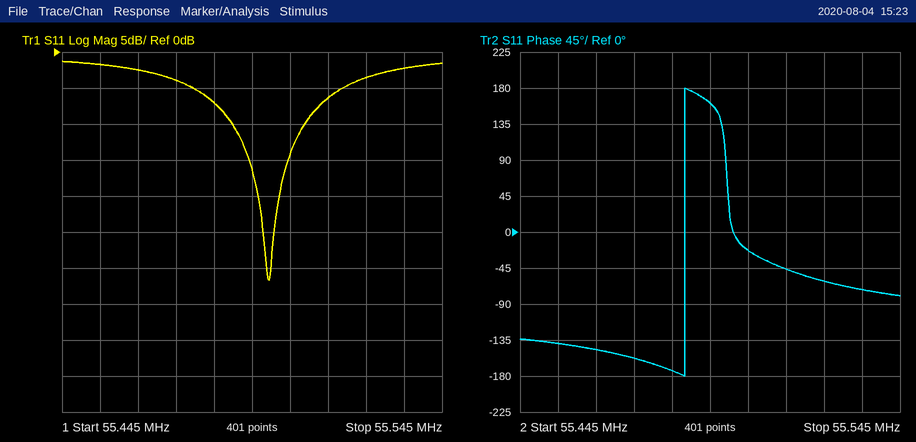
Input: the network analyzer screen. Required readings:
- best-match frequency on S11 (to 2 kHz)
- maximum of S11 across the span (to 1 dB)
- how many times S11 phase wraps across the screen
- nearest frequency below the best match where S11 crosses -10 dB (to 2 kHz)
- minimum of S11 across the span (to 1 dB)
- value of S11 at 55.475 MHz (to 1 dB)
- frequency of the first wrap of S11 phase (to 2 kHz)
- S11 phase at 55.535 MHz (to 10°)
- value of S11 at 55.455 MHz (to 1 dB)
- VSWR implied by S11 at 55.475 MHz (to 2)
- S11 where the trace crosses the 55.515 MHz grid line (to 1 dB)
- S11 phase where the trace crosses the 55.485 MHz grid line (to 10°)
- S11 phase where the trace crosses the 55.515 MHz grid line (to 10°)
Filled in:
55.500 MHz
-1 dB
1
55.490 MHz
-32 dB
-4 dB
55.488 MHz
-70°
-2 dB
4
-6 dB
-170°
-50°
